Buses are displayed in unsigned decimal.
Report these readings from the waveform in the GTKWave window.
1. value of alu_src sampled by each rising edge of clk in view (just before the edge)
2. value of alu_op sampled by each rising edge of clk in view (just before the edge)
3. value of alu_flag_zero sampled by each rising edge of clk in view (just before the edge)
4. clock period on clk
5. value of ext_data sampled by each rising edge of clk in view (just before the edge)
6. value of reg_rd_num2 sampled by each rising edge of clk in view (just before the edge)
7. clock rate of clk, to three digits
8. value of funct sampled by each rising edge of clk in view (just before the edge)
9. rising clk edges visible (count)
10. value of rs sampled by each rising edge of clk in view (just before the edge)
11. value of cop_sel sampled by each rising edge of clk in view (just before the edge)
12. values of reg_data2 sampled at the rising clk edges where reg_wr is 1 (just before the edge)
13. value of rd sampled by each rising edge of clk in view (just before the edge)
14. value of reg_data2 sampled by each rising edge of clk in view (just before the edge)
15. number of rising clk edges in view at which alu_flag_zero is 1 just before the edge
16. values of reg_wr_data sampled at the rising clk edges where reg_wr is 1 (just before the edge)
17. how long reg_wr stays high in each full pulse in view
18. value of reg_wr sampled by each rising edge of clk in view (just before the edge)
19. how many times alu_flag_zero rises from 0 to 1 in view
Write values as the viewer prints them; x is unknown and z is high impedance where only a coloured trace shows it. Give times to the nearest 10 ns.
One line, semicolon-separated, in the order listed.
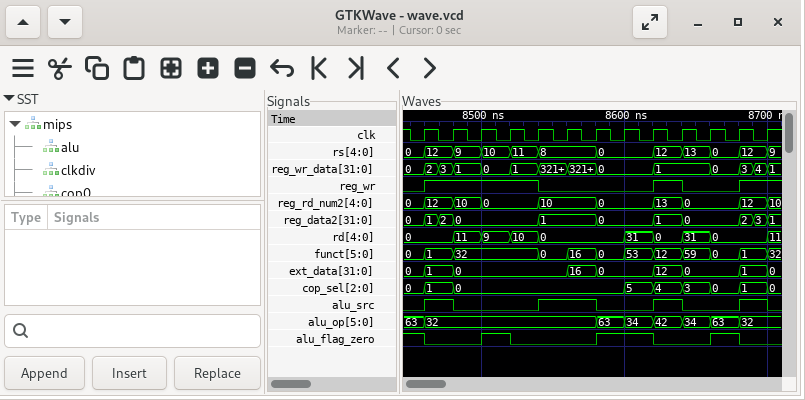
0 1 0 0 0 1 1 0 0 1 0 0 1; 63, 32, 32, 32, 32, 32, 32, 63, 34, 42, 34, 63, 32; 1 0 0 1 0 0 0 1 1 0 0 1 0; 20 ns; 0, 1, 0, 0, 0, 0, 16, 0, 0, 12, 0, 0, 1; 0, 12, 10, 0, 0, 10, 10, 0, 0, 13, 0, 0, 12; 50.0 MHz; 0, 1, 32, 32, 32, 0, 16, 0, 53, 12, 59, 0, 1; 13; 0, 12, 9, 10, 11, 8, 8, 0, 0, 12, 13, 0, 12; 0, 1, 0, 0, 0, 0, 0, 0, 5, 4, 3, 0, 1; 2, 0, 0, 0, 1, 3; 0, 0, 11, 9, 10, 0, 0, 0, 31, 0, 31, 0, 0; 0, 2, 0, 0, 0, 1, 1, 0, 0, 1, 0, 0, 3; 5; 3, 1, 0, 1, 1, 4; 80 ns, 20 ns; 0 1 1 1 1 0 0 0 0 1 0 0 1; 3
